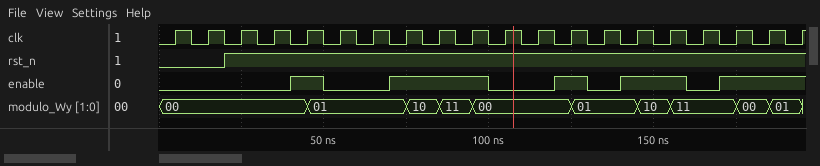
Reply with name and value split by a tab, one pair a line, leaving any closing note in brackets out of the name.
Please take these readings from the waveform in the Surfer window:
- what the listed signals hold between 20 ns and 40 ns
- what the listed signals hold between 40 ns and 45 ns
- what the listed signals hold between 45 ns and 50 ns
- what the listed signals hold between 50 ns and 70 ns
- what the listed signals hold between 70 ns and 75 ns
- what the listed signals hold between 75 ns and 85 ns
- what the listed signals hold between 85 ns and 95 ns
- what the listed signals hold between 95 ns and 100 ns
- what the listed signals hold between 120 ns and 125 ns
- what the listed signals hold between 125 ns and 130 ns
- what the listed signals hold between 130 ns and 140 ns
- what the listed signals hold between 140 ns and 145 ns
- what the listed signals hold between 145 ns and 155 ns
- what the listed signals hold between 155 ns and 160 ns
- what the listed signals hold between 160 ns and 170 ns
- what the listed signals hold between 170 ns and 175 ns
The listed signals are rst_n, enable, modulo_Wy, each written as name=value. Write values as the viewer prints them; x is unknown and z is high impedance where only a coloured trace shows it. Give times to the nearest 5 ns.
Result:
what the listed signals hold between 20 ns and 40 ns	rst_n=1, enable=0, modulo_Wy=00
what the listed signals hold between 40 ns and 45 ns	rst_n=1, enable=1, modulo_Wy=00
what the listed signals hold between 45 ns and 50 ns	rst_n=1, enable=1, modulo_Wy=01
what the listed signals hold between 50 ns and 70 ns	rst_n=1, enable=0, modulo_Wy=01
what the listed signals hold between 70 ns and 75 ns	rst_n=1, enable=1, modulo_Wy=01
what the listed signals hold between 75 ns and 85 ns	rst_n=1, enable=1, modulo_Wy=10
what the listed signals hold between 85 ns and 95 ns	rst_n=1, enable=1, modulo_Wy=11
what the listed signals hold between 95 ns and 100 ns	rst_n=1, enable=1, modulo_Wy=00
what the listed signals hold between 120 ns and 125 ns	rst_n=1, enable=1, modulo_Wy=00
what the listed signals hold between 125 ns and 130 ns	rst_n=1, enable=1, modulo_Wy=01
what the listed signals hold between 130 ns and 140 ns	rst_n=1, enable=0, modulo_Wy=01
what the listed signals hold between 140 ns and 145 ns	rst_n=1, enable=1, modulo_Wy=01
what the listed signals hold between 145 ns and 155 ns	rst_n=1, enable=1, modulo_Wy=10
what the listed signals hold between 155 ns and 160 ns	rst_n=1, enable=1, modulo_Wy=11
what the listed signals hold between 160 ns and 170 ns	rst_n=1, enable=0, modulo_Wy=11
what the listed signals hold between 170 ns and 175 ns	rst_n=1, enable=1, modulo_Wy=11
